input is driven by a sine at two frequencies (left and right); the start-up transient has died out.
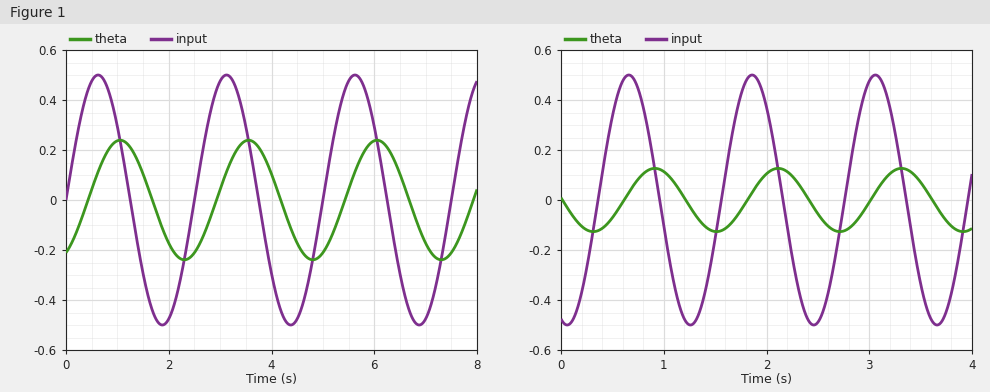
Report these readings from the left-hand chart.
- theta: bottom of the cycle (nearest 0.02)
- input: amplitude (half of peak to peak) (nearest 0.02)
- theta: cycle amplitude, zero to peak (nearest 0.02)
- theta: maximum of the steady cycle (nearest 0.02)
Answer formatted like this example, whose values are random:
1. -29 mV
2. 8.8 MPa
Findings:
1. -0.24
2. 0.50
3. 0.24
4. 0.24
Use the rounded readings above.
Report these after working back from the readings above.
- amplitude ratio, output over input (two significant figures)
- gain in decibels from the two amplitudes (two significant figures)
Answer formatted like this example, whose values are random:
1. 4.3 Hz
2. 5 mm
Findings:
1. 0.48
2. -6.4 dB
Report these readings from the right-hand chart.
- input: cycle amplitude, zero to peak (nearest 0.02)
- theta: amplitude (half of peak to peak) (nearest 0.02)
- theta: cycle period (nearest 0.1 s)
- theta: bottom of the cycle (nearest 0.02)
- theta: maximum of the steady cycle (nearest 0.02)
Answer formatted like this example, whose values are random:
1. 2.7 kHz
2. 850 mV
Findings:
1. 0.50
2. 0.12
3. 1.2 s
4. -0.12
5. 0.12
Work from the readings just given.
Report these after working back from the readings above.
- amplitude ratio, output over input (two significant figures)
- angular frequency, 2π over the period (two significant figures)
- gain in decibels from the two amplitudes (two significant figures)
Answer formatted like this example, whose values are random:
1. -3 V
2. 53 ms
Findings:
1. 0.24
2. 5.2 rad/s
3. -12 dB
